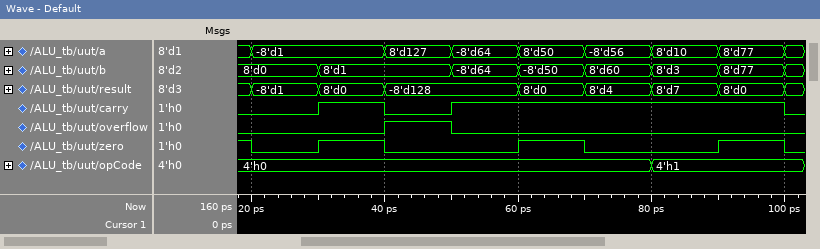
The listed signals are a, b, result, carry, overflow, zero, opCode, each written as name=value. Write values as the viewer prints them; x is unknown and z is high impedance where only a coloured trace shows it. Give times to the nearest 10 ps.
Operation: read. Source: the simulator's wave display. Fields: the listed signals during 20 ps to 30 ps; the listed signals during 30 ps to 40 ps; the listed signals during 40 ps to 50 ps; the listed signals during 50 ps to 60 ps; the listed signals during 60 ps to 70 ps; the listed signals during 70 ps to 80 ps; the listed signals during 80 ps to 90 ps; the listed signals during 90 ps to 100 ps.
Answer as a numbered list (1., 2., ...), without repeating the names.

1. a=-8'd1, b=8'd0, result=-8'd1, carry=0, overflow=0, zero=0, opCode=4'h0
2. a=-8'd1, b=8'd1, result=8'd0, carry=1, overflow=0, zero=1, opCode=4'h0
3. a=8'd127, b=8'd1, result=-8'd128, carry=0, overflow=1, zero=0, opCode=4'h0
4. a=-8'd64, b=-8'd64, result=-8'd128, carry=1, overflow=0, zero=0, opCode=4'h0
5. a=8'd50, b=-8'd50, result=8'd0, carry=1, overflow=0, zero=1, opCode=4'h0
6. a=-8'd56, b=8'd60, result=8'd4, carry=1, overflow=0, zero=0, opCode=4'h0
7. a=8'd10, b=8'd3, result=8'd7, carry=1, overflow=0, zero=0, opCode=4'h1
8. a=8'd77, b=8'd77, result=8'd0, carry=1, overflow=0, zero=1, opCode=4'h1
